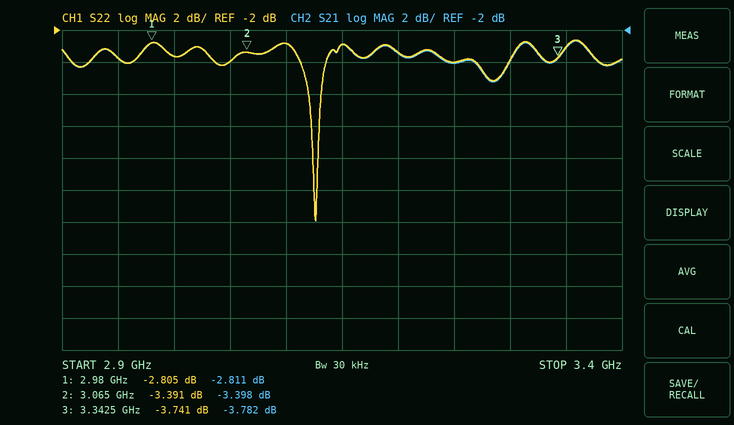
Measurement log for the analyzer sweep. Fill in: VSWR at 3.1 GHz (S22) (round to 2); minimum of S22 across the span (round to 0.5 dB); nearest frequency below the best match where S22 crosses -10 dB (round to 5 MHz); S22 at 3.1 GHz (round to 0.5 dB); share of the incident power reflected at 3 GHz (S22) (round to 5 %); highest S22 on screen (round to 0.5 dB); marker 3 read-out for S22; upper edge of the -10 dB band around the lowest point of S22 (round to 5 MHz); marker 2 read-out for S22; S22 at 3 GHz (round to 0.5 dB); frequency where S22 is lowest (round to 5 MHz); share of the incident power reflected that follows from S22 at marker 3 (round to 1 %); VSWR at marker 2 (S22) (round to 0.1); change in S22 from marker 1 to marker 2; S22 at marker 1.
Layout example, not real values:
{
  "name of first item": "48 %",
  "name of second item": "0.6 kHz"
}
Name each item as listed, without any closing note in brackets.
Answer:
{
  "VSWR at 3.1 GHz (S22)": "6",
  "minimum of S22 across the span": "-14.0 dB",
  "nearest frequency below the best match where S22 crosses -10 dB": "3.125 GHz",
  "S22 at 3.1 GHz": "-3.0 dB",
  "share of the incident power reflected at 3 GHz (S22)": "45 %",
  "highest S22 on screen": "-2.5 dB",
  "marker 3 read-out for S22": "-3.741 dB",
  "upper edge of the -10 dB band around the lowest point of S22": "3.130 GHz",
  "marker 2 read-out for S22": "-3.391 dB",
  "S22 at 3 GHz": "-3.5 dB",
  "frequency where S22 is lowest": "3.125 GHz",
  "share of the incident power reflected that follows from S22 at marker 3": "42 %",
  "VSWR at marker 2 (S22)": "5.2",
  "change in S22 from marker 1 to marker 2": "-0.586 dB",
  "S22 at marker 1": "-2.805 dB"
}
